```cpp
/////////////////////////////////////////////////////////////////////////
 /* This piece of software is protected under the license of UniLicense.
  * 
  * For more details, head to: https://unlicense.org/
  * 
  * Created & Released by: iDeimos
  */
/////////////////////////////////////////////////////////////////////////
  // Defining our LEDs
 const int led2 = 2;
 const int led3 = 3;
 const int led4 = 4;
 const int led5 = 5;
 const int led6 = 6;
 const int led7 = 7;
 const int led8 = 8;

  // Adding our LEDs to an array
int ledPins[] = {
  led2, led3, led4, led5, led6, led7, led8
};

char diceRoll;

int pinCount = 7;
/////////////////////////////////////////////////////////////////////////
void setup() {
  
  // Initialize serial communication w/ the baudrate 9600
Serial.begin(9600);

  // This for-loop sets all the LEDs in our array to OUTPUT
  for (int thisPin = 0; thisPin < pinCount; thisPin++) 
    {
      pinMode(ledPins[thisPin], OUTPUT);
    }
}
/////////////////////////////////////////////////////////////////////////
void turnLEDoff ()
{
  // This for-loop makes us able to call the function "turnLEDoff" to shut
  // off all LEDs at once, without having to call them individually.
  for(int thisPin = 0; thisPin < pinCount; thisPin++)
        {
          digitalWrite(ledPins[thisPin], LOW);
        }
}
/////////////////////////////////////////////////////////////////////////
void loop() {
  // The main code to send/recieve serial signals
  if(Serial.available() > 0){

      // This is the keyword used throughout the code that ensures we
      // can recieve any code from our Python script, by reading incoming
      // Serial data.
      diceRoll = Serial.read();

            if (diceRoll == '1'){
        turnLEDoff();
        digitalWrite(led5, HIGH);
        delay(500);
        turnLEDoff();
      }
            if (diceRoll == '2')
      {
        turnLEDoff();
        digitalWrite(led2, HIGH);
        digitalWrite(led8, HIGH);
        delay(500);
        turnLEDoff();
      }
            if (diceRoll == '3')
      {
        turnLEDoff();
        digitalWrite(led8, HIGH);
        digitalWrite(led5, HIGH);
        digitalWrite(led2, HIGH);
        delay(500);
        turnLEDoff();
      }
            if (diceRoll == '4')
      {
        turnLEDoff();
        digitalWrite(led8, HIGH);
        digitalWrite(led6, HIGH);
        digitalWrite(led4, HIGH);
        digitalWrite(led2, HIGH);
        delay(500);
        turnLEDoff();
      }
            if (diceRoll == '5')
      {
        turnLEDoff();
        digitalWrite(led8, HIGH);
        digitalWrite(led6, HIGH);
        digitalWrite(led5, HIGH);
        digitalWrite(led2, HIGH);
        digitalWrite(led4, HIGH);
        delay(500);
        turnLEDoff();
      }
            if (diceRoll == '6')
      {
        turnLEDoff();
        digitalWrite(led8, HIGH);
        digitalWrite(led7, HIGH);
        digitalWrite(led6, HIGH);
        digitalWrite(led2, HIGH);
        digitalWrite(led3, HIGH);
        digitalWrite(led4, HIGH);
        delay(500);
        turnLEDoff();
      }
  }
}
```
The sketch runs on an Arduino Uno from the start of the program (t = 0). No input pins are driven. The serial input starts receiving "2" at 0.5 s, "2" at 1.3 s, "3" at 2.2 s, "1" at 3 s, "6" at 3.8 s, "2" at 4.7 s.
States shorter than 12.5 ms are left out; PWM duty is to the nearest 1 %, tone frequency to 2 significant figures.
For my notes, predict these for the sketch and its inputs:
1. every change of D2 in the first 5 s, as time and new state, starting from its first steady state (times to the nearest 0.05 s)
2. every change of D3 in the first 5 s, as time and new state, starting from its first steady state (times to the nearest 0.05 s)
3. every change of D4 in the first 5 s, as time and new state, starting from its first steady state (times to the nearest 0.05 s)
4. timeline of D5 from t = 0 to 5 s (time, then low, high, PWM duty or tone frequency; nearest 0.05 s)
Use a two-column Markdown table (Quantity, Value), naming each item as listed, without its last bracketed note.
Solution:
| Quantity | Value |
|---|---|
| every change of D2 in the first 5 s, as time and new state, starting from its first steady state | 0 s low; 0.5 s high; 1 s low; 1.3 s high; 1.8 s low; 2.2 s high; 2.7 s low; 3.8 s high; 4.3 s low; 4.7 s high |
| every change of D3 in the first 5 s, as time and new state, starting from its first steady state | 0 s low; 3.8 s high; 4.3 s low |
| every change of D4 in the first 5 s, as time and new state, starting from its first steady state | 0 s low; 3.8 s high; 4.3 s low |
| timeline of D5 from t = 0 to 5 s | 0 s low; 2.2 s high; 2.7 s low; 3 s high; 3.5 s low |
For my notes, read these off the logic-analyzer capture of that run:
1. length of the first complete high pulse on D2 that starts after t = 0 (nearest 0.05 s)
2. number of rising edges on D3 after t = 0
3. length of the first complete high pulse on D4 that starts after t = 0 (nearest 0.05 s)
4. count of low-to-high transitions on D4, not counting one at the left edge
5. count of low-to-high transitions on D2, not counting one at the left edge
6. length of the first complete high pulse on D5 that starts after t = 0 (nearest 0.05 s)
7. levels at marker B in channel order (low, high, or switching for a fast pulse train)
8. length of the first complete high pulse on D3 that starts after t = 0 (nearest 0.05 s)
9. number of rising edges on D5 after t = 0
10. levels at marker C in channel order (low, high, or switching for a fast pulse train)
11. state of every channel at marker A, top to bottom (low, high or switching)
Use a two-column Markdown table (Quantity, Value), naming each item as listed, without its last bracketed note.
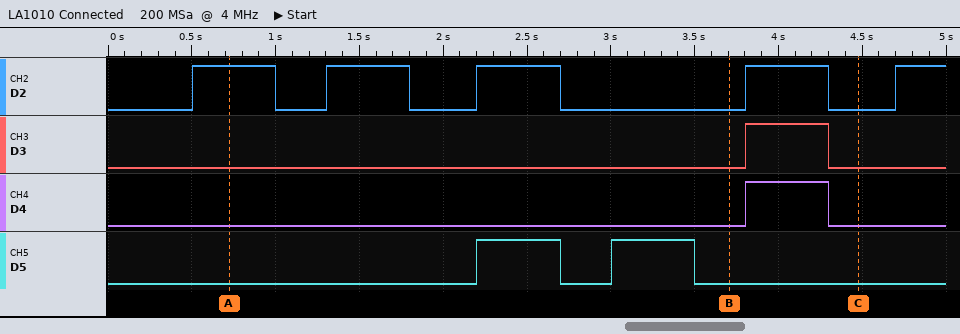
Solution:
| Quantity | Value |
|---|---|
| length of the first complete high pulse on D2 that starts after t = 0 | 0.50 s |
| number of rising edges on D3 after t = 0 | 1 |
| length of the first complete high pulse on D4 that starts after t = 0 | 0.50 s |
| count of low-to-high transitions on D4, not counting one at the left edge | 1 |
| count of low-to-high transitions on D2, not counting one at the left edge | 5 |
| length of the first complete high pulse on D5 that starts after t = 0 | 0.50 s |
| levels at marker B in channel order | D2 low, D3 low, D4 low, D5 low |
| length of the first complete high pulse on D3 that starts after t = 0 | 0.50 s |
| number of rising edges on D5 after t = 0 | 2 |
| levels at marker C in channel order | D2 low, D3 low, D4 low, D5 low |
| state of every channel at marker A, top to bottom | D2 high, D3 low, D4 low, D5 low |
